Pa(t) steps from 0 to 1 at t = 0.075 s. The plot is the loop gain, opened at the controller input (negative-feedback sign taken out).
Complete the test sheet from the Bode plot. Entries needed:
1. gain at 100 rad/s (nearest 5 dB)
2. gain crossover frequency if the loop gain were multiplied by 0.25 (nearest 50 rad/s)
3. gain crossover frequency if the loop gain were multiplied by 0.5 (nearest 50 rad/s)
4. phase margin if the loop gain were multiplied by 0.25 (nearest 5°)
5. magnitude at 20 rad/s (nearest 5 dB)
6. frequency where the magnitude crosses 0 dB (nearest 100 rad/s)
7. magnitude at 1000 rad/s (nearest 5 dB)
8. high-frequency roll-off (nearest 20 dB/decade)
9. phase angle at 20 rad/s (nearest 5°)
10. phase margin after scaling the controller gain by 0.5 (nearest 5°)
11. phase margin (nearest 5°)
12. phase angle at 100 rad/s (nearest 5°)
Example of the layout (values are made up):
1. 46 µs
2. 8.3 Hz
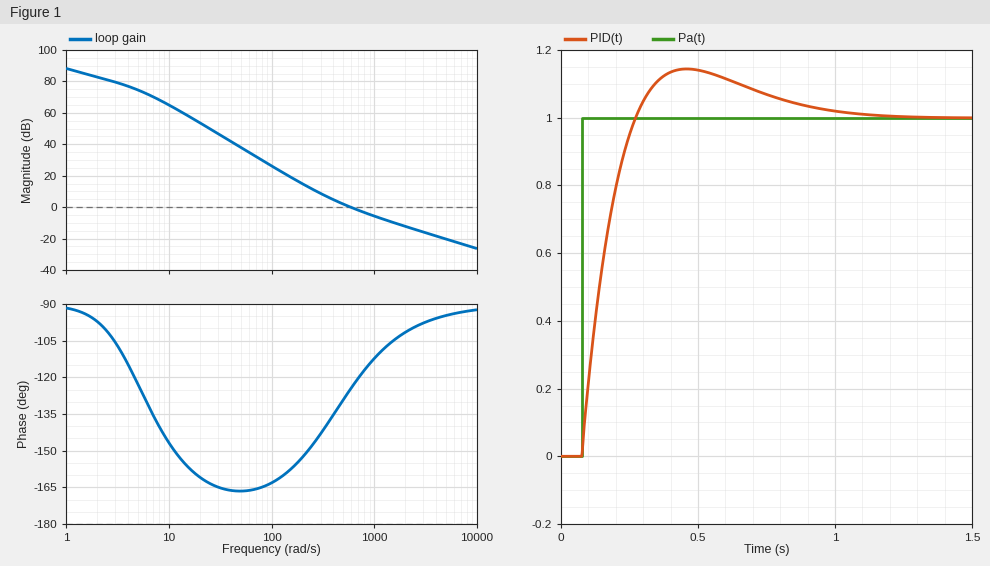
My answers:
1. 25 dB
2. 250 rad/s
3. 350 rad/s
4. 30°
5. 55 dB
6. 600 rad/s
7. -5 dB
8. -20 dB/decade
9. -160°
10. 40°
11. 55°
12. -165°
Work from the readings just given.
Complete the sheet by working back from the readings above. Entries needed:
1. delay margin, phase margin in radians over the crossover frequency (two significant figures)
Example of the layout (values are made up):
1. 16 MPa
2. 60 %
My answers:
1. 0.0016 s
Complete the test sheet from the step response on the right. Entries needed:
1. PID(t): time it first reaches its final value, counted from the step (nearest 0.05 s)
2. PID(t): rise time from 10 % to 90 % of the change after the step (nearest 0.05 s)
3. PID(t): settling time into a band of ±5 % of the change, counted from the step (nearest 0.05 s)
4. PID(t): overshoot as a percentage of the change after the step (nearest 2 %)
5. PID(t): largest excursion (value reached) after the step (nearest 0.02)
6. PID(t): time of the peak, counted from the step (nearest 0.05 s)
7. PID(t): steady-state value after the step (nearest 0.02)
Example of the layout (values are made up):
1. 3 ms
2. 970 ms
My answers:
1. 0.20 s
2. 0.15 s
3. 0.75 s
4. 14 %
5. 1.14
6. 0.40 s
7. 1.00
